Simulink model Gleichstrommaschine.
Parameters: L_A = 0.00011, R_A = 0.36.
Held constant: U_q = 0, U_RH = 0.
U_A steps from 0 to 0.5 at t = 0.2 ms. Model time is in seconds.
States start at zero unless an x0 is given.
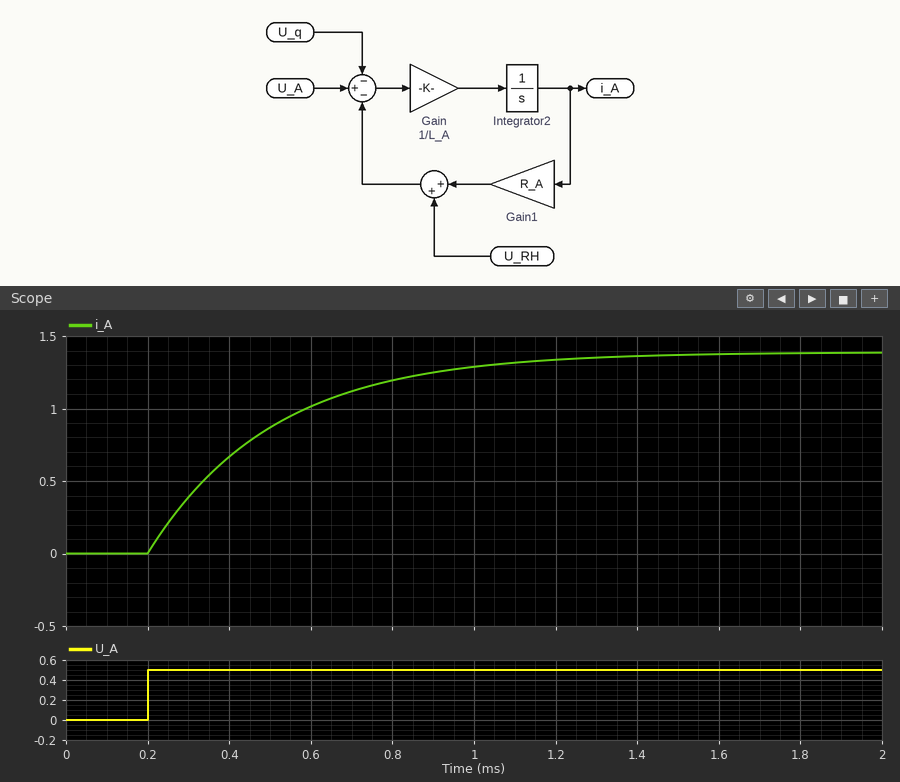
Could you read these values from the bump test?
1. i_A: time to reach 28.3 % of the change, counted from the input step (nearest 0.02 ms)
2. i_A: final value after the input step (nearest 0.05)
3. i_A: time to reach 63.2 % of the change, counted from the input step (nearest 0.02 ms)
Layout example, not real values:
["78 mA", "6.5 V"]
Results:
["0.10 ms", "1.40", "0.30 ms"]
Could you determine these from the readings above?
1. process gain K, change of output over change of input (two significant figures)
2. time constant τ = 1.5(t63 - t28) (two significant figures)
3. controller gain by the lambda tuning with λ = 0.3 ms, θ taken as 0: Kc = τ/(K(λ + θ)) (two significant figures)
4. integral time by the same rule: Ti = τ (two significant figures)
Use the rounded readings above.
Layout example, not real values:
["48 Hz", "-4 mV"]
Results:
["2.8", "0.30 ms", "0.36", "0.30 ms"]
